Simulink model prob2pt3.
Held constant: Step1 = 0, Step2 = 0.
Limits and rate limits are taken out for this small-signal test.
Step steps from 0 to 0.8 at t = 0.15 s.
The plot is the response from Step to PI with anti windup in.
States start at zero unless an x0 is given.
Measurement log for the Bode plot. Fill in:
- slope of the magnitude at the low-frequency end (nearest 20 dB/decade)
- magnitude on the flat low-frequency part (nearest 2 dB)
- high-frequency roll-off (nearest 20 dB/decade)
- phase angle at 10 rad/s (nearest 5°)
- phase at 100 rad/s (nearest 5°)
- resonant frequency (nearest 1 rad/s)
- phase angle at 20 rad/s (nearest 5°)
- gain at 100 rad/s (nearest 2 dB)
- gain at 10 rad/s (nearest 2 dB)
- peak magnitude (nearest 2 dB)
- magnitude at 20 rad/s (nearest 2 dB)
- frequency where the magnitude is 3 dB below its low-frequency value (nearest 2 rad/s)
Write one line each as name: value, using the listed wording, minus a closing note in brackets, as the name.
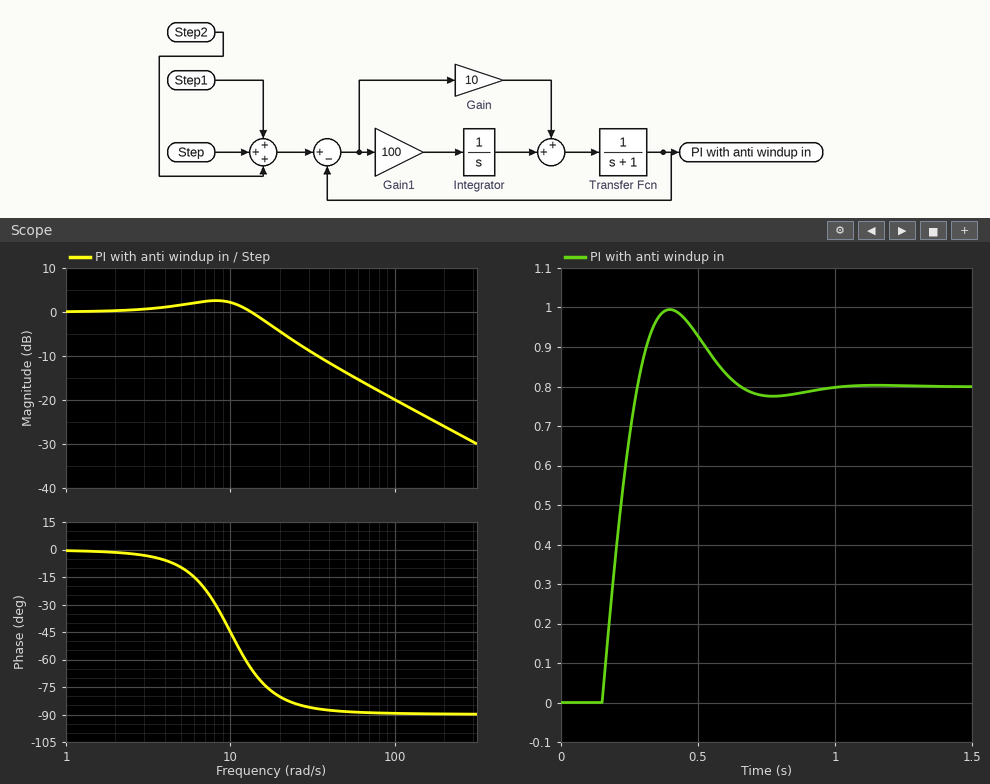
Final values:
slope of the magnitude at the low-frequency end: 0 dB/decade
magnitude on the flat low-frequency part: 0 dB
high-frequency roll-off: -20 dB/decade
phase angle at 10 rad/s: -45°
phase at 100 rad/s: -90°
resonant frequency: 8 rad/s
phase angle at 20 rad/s: -80°
gain at 100 rad/s: -20 dB
gain at 10 rad/s: 2 dB
peak magnitude: 2 dB
magnitude at 20 rad/s: -4 dB
frequency where the magnitude is 3 dB below its low-frequency value: 18 rad/s
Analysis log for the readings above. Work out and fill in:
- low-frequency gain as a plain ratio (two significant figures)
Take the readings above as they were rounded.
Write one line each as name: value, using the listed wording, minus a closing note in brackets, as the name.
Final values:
low-frequency gain as a plain ratio: 1.0
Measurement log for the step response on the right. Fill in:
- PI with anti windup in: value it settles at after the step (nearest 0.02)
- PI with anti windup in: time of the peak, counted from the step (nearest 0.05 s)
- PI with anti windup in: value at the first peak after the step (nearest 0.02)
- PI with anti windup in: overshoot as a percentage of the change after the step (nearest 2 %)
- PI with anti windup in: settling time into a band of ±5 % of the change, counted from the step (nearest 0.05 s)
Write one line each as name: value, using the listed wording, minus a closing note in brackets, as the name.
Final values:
PI with anti windup in: value it settles at after the step: 0.80
PI with anti windup in: time of the peak, counted from the step: 0.25 s
PI with anti windup in: value at the first peak after the step: 1.00
PI with anti windup in: overshoot as a percentage of the change after the step: 24 %
PI with anti windup in: settling time into a band of ±5 % of the change, counted from the step: 0.45 s
